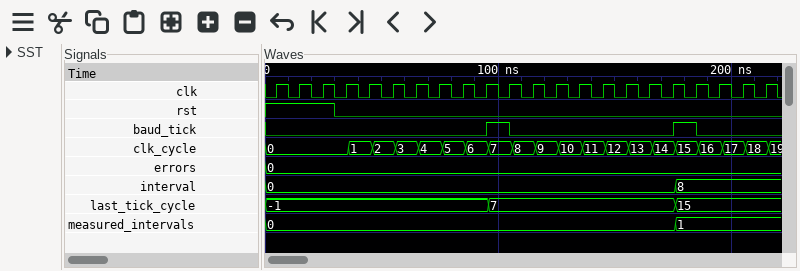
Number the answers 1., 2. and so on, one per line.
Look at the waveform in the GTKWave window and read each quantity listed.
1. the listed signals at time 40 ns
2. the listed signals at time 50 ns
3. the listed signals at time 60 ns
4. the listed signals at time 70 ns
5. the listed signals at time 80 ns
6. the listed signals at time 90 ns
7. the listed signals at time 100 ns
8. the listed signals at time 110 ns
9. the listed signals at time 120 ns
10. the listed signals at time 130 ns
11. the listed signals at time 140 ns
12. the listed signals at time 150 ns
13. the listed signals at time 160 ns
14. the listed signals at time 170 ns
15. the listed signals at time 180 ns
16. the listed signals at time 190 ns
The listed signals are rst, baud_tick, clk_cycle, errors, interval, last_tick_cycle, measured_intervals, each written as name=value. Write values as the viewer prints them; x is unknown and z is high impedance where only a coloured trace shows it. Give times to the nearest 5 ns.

1. rst=0, baud_tick=0, clk_cycle=1, errors=0, interval=0, last_tick_cycle=-1, measured_intervals=0
2. rst=0, baud_tick=0, clk_cycle=2, errors=0, interval=0, last_tick_cycle=-1, measured_intervals=0
3. rst=0, baud_tick=0, clk_cycle=3, errors=0, interval=0, last_tick_cycle=-1, measured_intervals=0
4. rst=0, baud_tick=0, clk_cycle=4, errors=0, interval=0, last_tick_cycle=-1, measured_intervals=0
5. rst=0, baud_tick=0, clk_cycle=5, errors=0, interval=0, last_tick_cycle=-1, measured_intervals=0
6. rst=0, baud_tick=0, clk_cycle=6, errors=0, interval=0, last_tick_cycle=-1, measured_intervals=0
7. rst=0, baud_tick=1, clk_cycle=7, errors=0, interval=0, last_tick_cycle=7, measured_intervals=0
8. rst=0, baud_tick=0, clk_cycle=8, errors=0, interval=0, last_tick_cycle=7, measured_intervals=0
9. rst=0, baud_tick=0, clk_cycle=9, errors=0, interval=0, last_tick_cycle=7, measured_intervals=0
10. rst=0, baud_tick=0, clk_cycle=10, errors=0, interval=0, last_tick_cycle=7, measured_intervals=0
11. rst=0, baud_tick=0, clk_cycle=11, errors=0, interval=0, last_tick_cycle=7, measured_intervals=0
12. rst=0, baud_tick=0, clk_cycle=12, errors=0, interval=0, last_tick_cycle=7, measured_intervals=0
13. rst=0, baud_tick=0, clk_cycle=13, errors=0, interval=0, last_tick_cycle=7, measured_intervals=0
14. rst=0, baud_tick=0, clk_cycle=14, errors=0, interval=0, last_tick_cycle=7, measured_intervals=0
15. rst=0, baud_tick=1, clk_cycle=15, errors=0, interval=8, last_tick_cycle=15, measured_intervals=1
16. rst=0, baud_tick=0, clk_cycle=16, errors=0, interval=8, last_tick_cycle=15, measured_intervals=1
